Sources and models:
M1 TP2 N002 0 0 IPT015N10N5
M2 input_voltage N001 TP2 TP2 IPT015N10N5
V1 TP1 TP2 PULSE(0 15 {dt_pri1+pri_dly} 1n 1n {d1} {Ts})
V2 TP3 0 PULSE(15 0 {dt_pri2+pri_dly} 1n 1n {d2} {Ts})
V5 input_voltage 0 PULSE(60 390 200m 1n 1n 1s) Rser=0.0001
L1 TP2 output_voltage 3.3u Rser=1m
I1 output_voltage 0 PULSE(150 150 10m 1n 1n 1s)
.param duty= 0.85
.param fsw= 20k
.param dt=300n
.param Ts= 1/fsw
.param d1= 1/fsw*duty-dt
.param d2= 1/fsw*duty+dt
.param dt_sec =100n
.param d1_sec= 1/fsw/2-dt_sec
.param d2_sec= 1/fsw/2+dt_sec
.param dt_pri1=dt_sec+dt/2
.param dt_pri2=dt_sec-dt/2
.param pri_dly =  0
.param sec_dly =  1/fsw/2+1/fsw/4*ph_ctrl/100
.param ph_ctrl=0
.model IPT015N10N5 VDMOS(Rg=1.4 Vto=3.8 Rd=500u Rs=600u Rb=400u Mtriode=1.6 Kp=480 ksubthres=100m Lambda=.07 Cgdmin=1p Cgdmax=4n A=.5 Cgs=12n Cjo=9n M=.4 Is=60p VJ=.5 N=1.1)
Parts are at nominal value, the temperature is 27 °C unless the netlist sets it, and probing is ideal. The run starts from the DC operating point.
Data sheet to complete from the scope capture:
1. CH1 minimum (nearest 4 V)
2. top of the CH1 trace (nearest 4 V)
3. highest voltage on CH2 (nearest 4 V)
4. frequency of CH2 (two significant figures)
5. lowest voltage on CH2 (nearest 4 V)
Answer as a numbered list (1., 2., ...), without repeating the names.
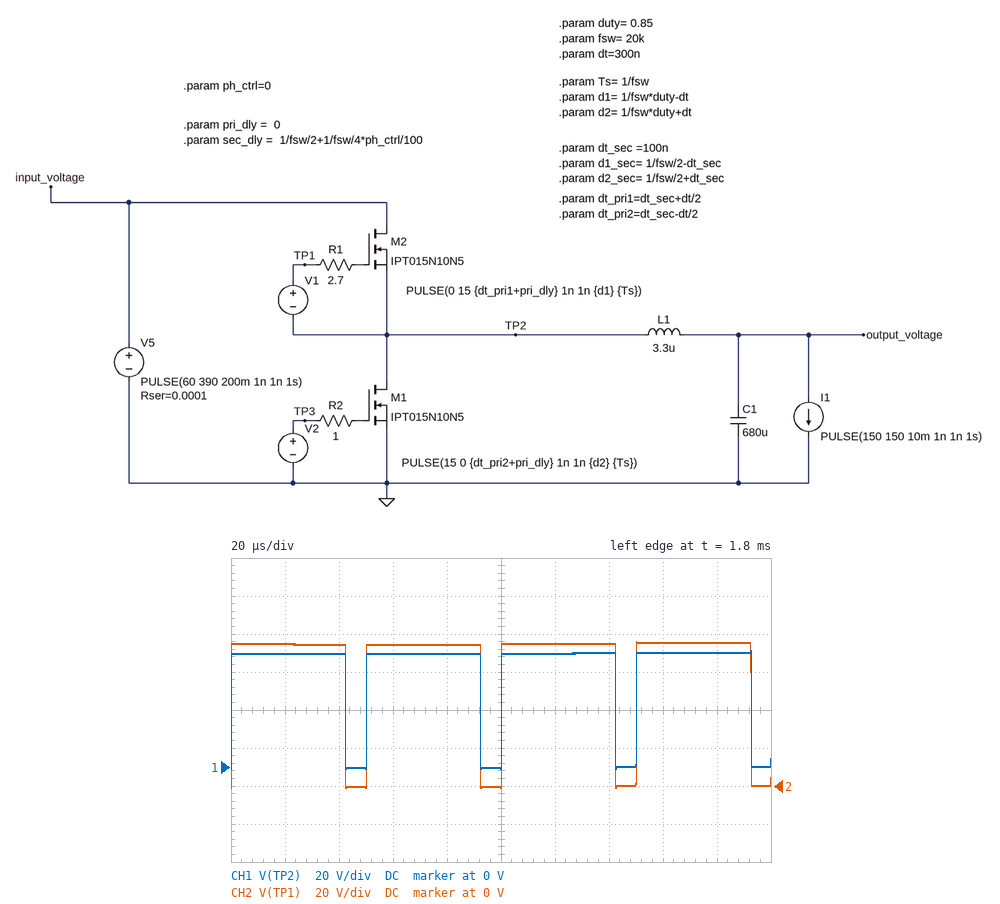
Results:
1. 0 V
2. 60 V
3. 76 V
4. 20 kHz
5. 0 V
